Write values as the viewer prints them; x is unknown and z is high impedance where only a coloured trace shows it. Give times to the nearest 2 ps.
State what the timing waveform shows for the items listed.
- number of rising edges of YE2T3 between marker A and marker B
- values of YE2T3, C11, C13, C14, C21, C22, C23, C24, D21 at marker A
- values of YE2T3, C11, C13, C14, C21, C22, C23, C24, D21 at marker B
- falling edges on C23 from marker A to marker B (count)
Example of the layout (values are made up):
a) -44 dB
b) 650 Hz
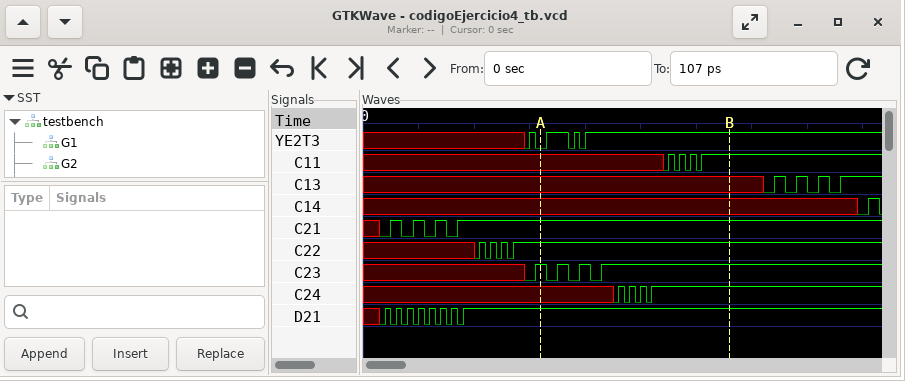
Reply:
a) 3
b) YE2T3=0, C11=x, C13=x, C14=x, C21=1, C22=1, C23=1, C24=x, D21=1
c) YE2T3=1, C11=1, C13=x, C14=x, C21=1, C22=1, C23=1, C24=1, D21=1
d) 3
